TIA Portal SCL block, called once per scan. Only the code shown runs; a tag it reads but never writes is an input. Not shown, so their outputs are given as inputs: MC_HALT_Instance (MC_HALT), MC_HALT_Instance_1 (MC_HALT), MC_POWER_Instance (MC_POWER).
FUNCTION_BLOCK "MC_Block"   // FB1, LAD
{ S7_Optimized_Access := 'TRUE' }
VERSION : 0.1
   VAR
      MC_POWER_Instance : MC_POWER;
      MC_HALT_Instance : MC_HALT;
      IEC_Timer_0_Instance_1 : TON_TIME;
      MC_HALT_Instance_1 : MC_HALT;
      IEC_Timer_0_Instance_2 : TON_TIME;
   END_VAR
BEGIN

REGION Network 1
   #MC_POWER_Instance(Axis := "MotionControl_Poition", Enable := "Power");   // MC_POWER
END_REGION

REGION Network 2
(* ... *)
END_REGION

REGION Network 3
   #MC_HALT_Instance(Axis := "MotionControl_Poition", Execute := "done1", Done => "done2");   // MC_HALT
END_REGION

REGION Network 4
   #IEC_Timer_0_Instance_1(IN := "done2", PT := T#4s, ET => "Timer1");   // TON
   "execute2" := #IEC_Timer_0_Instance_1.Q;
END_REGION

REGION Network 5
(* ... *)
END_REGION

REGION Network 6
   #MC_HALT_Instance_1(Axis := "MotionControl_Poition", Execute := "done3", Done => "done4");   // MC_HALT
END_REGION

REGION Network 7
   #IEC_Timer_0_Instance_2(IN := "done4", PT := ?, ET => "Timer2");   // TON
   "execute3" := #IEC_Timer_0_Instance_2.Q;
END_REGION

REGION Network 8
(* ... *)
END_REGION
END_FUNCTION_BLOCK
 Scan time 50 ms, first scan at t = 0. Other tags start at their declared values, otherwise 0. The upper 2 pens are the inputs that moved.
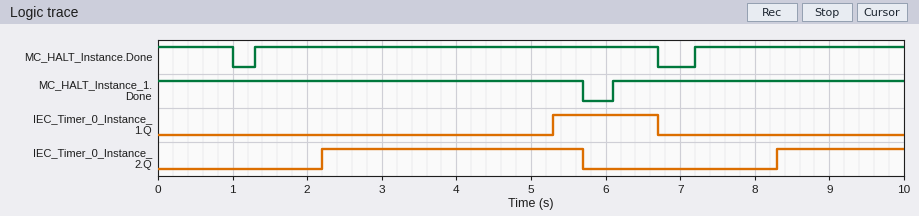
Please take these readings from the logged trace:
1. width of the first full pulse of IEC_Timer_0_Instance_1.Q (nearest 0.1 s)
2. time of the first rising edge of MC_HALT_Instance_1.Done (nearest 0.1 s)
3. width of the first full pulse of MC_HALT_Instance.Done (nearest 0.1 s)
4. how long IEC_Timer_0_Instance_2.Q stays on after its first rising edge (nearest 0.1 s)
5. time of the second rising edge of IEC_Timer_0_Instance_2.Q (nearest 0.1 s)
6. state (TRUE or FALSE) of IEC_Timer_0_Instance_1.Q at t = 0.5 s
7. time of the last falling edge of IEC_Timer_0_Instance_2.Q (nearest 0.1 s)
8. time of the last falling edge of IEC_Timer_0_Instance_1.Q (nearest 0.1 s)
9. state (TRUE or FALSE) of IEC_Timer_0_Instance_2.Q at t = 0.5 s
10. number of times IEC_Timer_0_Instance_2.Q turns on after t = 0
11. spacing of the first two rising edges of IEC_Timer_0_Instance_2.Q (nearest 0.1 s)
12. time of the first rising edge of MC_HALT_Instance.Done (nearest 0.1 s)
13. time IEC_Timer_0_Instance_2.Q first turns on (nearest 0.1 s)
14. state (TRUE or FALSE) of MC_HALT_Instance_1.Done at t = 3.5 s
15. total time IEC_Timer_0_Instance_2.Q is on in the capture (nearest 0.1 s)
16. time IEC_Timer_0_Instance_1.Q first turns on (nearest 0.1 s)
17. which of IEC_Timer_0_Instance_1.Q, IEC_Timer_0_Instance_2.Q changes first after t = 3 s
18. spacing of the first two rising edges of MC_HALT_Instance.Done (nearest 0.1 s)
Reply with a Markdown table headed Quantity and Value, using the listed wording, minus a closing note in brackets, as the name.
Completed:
| Quantity | Value |
|---|---|
| width of the first full pulse of IEC_Timer_0_Instance_1.Q | 1.4 s |
| time of the first rising edge of MC_HALT_Instance_1.Done | 6.1 s |
| width of the first full pulse of MC_HALT_Instance.Done | 5.4 s |
| how long IEC_Timer_0_Instance_2.Q stays on after its first rising edge | 3.5 s |
| time of the second rising edge of IEC_Timer_0_Instance_2.Q | 8.3 s |
| state (TRUE or FALSE) of IEC_Timer_0_Instance_1.Q at t = 0.5 s | FALSE |
| time of the last falling edge of IEC_Timer_0_Instance_2.Q | 5.7 s |
| time of the last falling edge of IEC_Timer_0_Instance_1.Q | 6.7 s |
| state (TRUE or FALSE) of IEC_Timer_0_Instance_2.Q at t = 0.5 s | FALSE |
| number of times IEC_Timer_0_Instance_2.Q turns on after t = 0 | 2 |
| spacing of the first two rising edges of IEC_Timer_0_Instance_2.Q | 6.1 s |
| time of the first rising edge of MC_HALT_Instance.Done | 1.3 s |
| time IEC_Timer_0_Instance_2.Q first turns on | 2.2 s |
| state (TRUE or FALSE) of MC_HALT_Instance_1.Done at t = 3.5 s | TRUE |
| total time IEC_Timer_0_Instance_2.Q is on in the capture | 5.2 s |
| time IEC_Timer_0_Instance_1.Q first turns on | 5.3 s |
| which of IEC_Timer_0_Instance_1.Q, IEC_Timer_0_Instance_2.Q changes first after t = 3 s | IEC_Timer_0_Instance_1.Q |
| spacing of the first two rising edges of MC_HALT_Instance.Done | 5.9 s |
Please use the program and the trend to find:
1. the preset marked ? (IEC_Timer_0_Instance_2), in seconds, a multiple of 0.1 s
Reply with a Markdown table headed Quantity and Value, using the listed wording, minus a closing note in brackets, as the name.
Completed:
| Quantity | Value |
|---|---|
| the preset marked ? (IEC_Timer_0_Instance_2), in seconds, a multiple of 0.1 s | 2.2 s |
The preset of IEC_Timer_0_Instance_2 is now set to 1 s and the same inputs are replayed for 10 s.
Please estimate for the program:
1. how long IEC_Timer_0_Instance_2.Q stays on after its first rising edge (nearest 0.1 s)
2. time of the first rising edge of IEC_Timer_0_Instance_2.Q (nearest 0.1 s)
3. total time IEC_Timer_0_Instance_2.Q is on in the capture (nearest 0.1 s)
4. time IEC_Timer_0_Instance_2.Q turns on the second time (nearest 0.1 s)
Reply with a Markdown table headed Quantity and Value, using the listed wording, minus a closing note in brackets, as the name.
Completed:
| Quantity | Value |
|---|---|
| how long IEC_Timer_0_Instance_2.Q stays on after its first rising edge | 4.7 s |
| time of the first rising edge of IEC_Timer_0_Instance_2.Q | 1.0 s |
| total time IEC_Timer_0_Instance_2.Q is on in the capture | 7.6 s |
| time IEC_Timer_0_Instance_2.Q turns on the second time | 7.1 s |
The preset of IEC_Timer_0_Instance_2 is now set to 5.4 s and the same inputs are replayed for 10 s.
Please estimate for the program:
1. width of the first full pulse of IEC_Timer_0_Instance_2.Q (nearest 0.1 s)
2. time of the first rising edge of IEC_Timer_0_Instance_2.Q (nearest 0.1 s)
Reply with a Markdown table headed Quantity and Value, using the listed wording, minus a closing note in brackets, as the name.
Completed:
| Quantity | Value |
|---|---|
| width of the first full pulse of IEC_Timer_0_Instance_2.Q | 0.3 s |
| time of the first rising edge of IEC_Timer_0_Instance_2.Q | 5.4 s |
